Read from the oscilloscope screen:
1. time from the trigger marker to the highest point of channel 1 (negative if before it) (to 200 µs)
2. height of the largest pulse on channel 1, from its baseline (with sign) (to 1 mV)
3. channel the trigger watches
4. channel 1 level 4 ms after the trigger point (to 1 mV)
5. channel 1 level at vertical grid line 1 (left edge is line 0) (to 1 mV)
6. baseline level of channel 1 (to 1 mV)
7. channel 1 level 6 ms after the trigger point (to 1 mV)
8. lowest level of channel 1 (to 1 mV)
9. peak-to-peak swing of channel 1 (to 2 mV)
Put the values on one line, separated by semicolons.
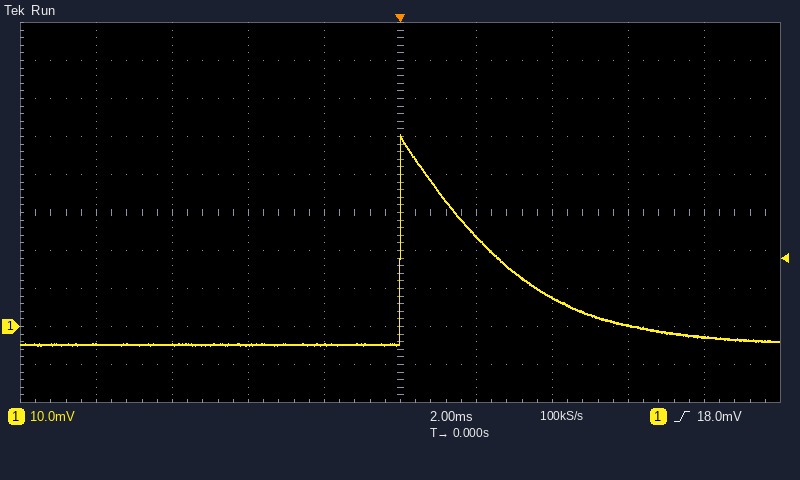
0.0 ms; +55 mV; channel 1; 8 mV; -5 mV; -5 mV; 0 mV; -5 mV; 56 mV
